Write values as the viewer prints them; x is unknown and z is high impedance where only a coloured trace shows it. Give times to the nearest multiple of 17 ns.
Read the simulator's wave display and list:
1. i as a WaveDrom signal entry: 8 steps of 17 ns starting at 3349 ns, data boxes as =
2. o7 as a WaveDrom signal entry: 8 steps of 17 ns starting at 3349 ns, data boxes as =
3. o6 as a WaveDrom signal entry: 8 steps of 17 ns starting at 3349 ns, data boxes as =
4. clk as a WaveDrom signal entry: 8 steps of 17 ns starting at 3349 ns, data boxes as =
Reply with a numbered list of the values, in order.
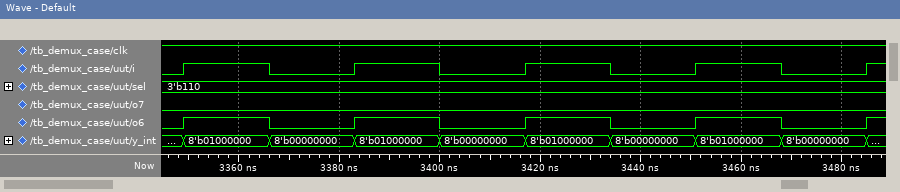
1. {name: 'i', wave: '10101010'}
2. {name: 'o7', wave: '0.......'}
3. {name: 'o6', wave: '10101010'}
4. {name: 'clk', wave: '1.......'}
